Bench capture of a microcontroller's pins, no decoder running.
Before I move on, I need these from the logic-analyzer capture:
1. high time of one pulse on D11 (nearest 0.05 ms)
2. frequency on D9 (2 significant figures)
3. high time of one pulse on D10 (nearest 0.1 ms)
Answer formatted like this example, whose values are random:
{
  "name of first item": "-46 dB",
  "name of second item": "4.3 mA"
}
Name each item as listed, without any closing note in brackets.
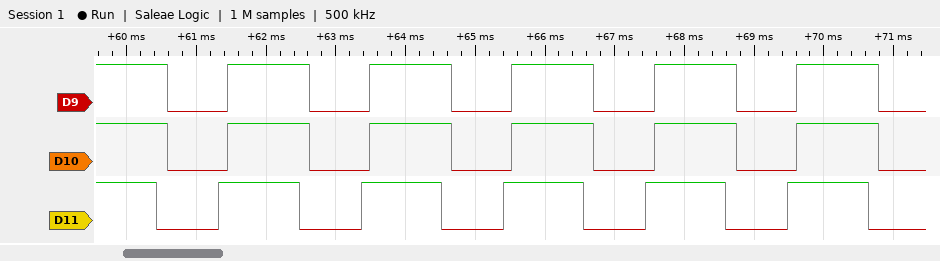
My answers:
{
  "high time of one pulse on D11": "1.15 ms",
  "frequency on D9": "490 Hz",
  "high time of one pulse on D10": "1.2 ms"
}
